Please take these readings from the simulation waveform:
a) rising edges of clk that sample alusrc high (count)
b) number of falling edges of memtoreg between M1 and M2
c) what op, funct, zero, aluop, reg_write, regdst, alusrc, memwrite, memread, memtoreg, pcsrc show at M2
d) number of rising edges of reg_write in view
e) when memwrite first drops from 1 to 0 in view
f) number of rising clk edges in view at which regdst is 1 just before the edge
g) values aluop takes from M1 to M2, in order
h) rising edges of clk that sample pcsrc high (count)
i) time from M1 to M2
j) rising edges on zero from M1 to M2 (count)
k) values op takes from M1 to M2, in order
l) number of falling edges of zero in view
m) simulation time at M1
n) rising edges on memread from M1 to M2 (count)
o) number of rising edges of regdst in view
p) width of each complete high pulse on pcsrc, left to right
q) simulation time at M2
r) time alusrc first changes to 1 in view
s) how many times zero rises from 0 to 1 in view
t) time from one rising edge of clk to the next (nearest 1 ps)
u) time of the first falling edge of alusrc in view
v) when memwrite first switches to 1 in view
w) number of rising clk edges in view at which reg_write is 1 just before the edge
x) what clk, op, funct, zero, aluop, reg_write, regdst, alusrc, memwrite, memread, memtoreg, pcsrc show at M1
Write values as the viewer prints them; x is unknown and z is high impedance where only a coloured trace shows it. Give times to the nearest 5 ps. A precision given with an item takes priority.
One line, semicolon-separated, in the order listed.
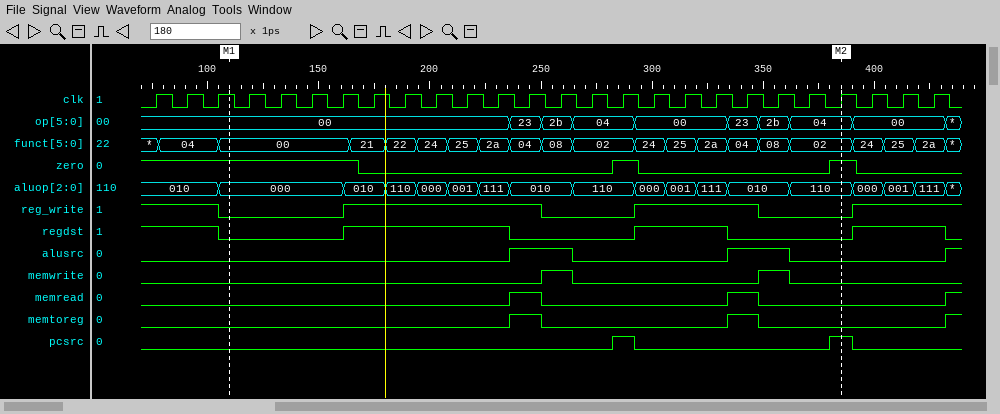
4; 2; op=04, funct=02, zero=1, aluop=110, reg_write=0, regdst=0, alusrc=0, memwrite=0, memread=0, memtoreg=0, pcsrc=1; 3; 265 ps; 14; 000, 010, 110, 000, 001, 111, 010, 110, 000, 001, 111, 010, 110; 2; 275 ps; 2; 00, 23, 2b, 04, 00, 23, 2b, 04; 3; 110 ps; 2; 3; 10 ps, 10 ps; 385 ps; 235 ps; 2; 14 ps; 265 ps; 250 ps; 16; clk=1, op=00, funct=00, zero=1, aluop=000, reg_write=0, regdst=0, alusrc=0, memwrite=0, memread=0, memtoreg=0, pcsrc=0
